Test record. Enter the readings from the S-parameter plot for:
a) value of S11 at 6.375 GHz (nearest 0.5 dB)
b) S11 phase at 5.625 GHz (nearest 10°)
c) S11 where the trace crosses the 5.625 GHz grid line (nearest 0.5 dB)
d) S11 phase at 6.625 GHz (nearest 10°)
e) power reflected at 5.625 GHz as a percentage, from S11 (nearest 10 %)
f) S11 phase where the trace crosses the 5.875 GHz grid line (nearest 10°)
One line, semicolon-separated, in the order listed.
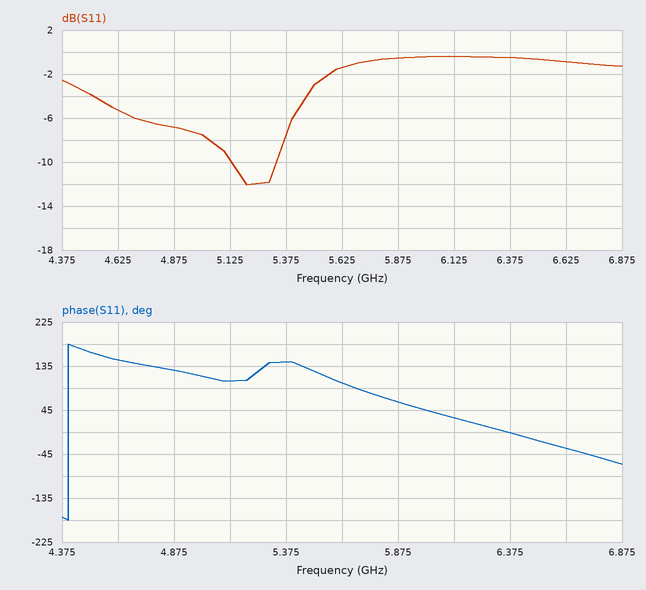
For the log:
-0.5 dB; 100°; -1.5 dB; -30°; 70 %; 60°
